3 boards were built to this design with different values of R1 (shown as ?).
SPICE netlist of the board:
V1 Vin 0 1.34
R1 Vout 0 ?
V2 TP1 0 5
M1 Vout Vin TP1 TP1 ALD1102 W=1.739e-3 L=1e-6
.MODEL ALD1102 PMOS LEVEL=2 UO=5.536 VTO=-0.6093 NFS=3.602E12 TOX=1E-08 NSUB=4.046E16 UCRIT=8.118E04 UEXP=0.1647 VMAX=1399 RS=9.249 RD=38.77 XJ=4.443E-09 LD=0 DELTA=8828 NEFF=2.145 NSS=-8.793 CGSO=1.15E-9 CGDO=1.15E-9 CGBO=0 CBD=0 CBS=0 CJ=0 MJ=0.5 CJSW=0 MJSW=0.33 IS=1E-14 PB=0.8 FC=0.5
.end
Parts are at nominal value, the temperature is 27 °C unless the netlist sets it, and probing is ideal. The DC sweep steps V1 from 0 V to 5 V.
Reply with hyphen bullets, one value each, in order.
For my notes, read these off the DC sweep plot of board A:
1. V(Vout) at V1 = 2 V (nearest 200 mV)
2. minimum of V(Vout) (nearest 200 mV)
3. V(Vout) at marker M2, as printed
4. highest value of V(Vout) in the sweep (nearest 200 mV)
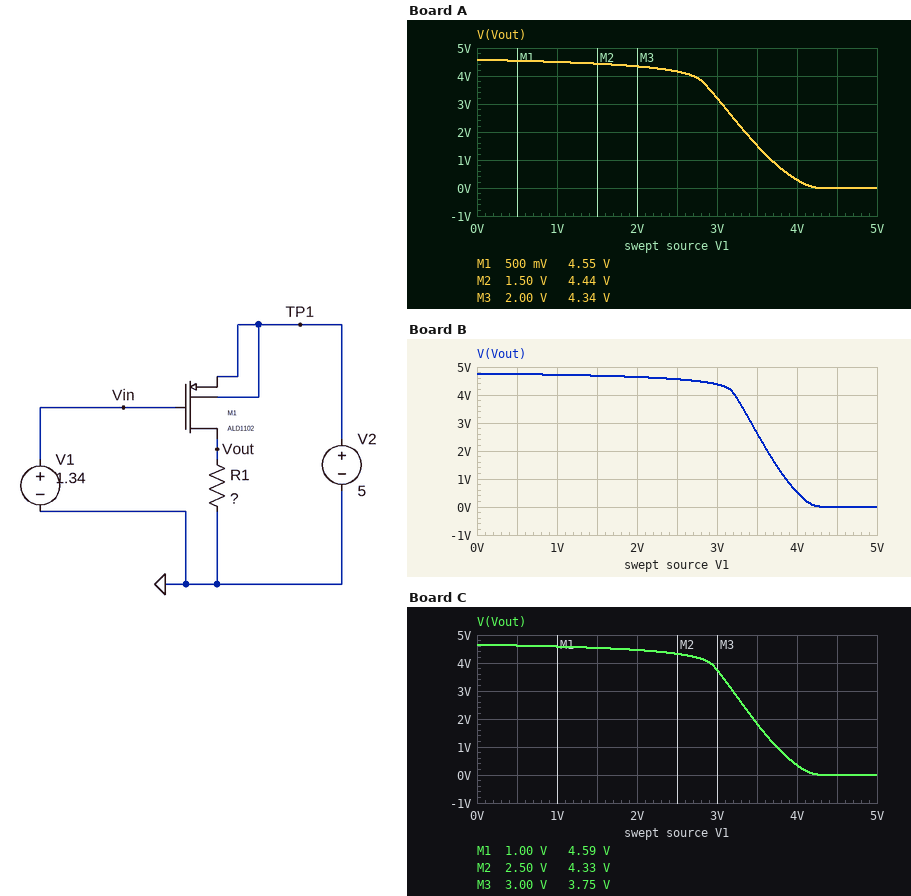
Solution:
- 4.4 V
- 0 V
- 4.44 V
- 4.6 V
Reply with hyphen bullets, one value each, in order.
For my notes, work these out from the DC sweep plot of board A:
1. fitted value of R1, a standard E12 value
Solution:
- 1.8 kΩ
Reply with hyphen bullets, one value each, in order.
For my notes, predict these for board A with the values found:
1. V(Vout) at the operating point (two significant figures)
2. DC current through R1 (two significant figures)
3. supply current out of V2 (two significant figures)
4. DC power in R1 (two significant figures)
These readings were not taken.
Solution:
- 4.5 V
- 2.5 mA
- 2.5 mA
- 11 mW
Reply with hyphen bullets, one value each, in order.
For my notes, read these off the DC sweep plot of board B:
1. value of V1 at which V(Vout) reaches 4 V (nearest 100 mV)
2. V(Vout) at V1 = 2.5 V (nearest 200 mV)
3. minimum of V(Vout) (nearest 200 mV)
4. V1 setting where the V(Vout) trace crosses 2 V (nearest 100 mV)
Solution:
- 3.2 V
- 4.6 V
- 0 V
- 3.6 V
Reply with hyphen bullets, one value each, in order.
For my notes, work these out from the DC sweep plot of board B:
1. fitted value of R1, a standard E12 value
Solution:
- 3.3 kΩ
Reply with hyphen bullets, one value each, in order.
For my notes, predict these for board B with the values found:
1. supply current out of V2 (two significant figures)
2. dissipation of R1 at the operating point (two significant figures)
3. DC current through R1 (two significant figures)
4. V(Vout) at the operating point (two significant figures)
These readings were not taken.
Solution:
- 1.4 mA
- 6.7 mW
- 1.4 mA
- 4.7 V
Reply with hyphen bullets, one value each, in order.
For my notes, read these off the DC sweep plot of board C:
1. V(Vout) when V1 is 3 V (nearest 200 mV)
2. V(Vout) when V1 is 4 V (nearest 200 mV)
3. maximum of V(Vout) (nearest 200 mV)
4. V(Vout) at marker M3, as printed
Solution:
- 3.8 V
- 400 mV
- 4.6 V
- 3.75 V
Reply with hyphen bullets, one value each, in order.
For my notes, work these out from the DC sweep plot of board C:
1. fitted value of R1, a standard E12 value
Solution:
- 2.2 kΩ
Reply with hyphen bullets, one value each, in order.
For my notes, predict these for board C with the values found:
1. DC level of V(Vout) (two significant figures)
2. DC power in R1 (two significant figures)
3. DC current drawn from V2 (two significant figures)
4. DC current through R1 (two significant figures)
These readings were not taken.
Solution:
- 4.6 V
- 9.4 mW
- 2.1 mA
- 2.1 mA
